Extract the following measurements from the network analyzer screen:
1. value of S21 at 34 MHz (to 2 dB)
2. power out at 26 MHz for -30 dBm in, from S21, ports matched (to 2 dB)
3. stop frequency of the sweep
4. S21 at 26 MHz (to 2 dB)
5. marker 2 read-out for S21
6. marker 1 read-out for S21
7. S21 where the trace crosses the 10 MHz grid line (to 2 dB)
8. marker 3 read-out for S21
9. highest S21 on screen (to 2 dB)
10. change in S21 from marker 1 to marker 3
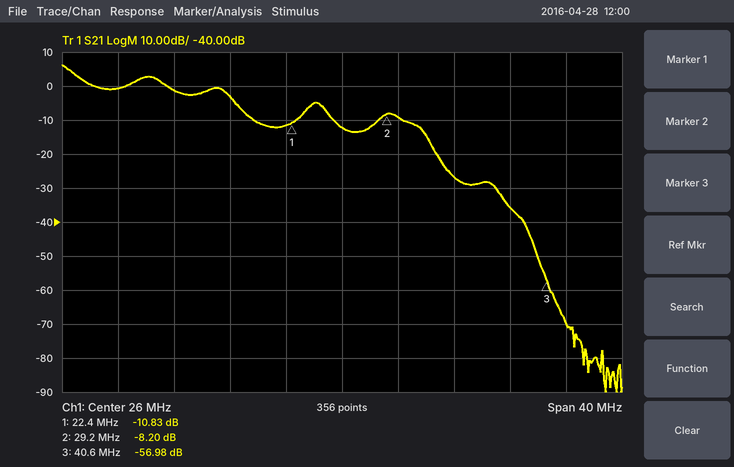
-26 dB
-42 dBm
46 MHz
-12 dB
-8.20 dB
-10.83 dB
0 dB
-56.98 dB
6 dB
-46.15 dB
